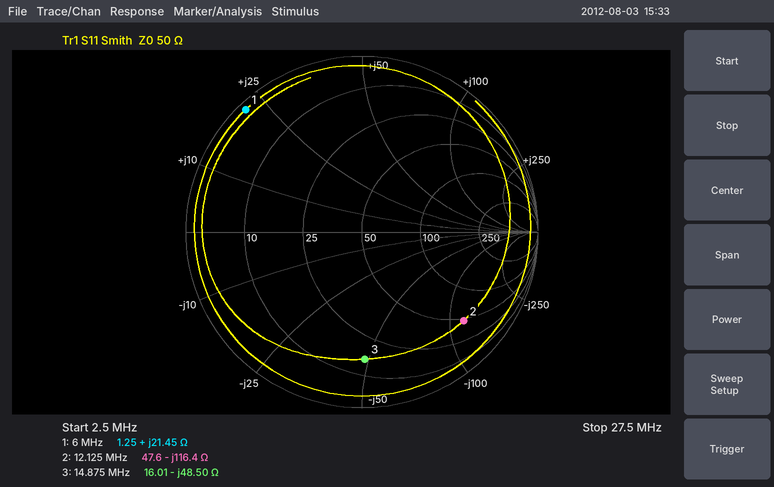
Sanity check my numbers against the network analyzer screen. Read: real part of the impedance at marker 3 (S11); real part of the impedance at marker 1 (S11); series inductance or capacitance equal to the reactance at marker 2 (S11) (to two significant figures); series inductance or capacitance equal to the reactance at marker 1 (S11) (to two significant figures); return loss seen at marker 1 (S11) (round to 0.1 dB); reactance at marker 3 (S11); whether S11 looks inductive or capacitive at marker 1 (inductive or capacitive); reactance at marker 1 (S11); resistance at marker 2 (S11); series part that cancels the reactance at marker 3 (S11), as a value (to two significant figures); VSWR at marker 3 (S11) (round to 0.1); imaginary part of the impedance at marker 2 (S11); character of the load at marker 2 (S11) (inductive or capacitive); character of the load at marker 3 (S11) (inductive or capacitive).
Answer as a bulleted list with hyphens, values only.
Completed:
- 16.01 Ω
- 1.25 Ω
- 110 pF
- 570 nH
- 0.4 dB
- -48.50 Ω
- inductive
- +21.45 Ω
- 47.6 Ω
- 520 nH
- 6.2
- -116.4 Ω
- capacitive
- capacitive
